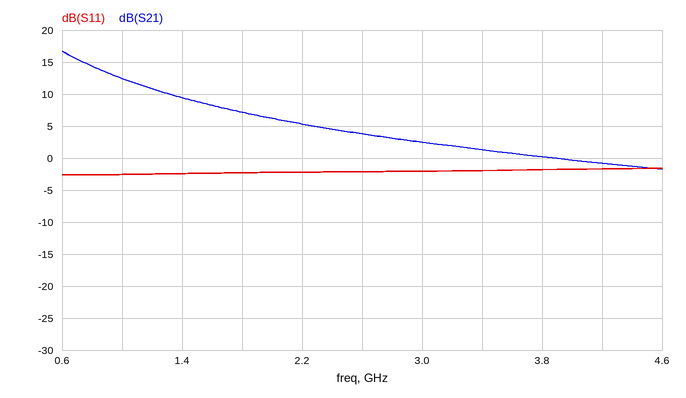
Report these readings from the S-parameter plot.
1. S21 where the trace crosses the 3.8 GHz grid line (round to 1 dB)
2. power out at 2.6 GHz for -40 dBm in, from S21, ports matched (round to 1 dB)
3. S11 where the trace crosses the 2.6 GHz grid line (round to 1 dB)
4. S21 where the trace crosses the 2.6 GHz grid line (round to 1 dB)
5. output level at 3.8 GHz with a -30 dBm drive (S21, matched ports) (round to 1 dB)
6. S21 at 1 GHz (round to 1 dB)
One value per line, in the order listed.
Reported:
0 dB
-36 dBm
-2 dB
4 dB
-30 dBm
12 dB
